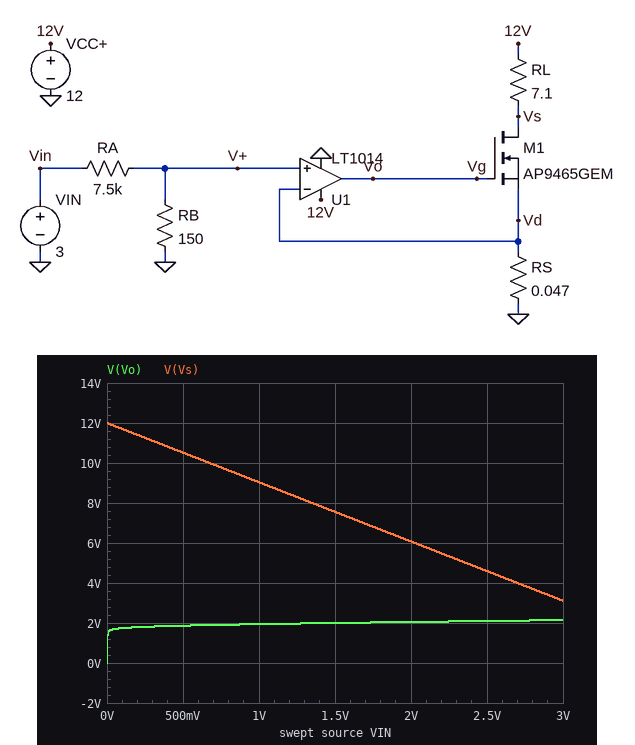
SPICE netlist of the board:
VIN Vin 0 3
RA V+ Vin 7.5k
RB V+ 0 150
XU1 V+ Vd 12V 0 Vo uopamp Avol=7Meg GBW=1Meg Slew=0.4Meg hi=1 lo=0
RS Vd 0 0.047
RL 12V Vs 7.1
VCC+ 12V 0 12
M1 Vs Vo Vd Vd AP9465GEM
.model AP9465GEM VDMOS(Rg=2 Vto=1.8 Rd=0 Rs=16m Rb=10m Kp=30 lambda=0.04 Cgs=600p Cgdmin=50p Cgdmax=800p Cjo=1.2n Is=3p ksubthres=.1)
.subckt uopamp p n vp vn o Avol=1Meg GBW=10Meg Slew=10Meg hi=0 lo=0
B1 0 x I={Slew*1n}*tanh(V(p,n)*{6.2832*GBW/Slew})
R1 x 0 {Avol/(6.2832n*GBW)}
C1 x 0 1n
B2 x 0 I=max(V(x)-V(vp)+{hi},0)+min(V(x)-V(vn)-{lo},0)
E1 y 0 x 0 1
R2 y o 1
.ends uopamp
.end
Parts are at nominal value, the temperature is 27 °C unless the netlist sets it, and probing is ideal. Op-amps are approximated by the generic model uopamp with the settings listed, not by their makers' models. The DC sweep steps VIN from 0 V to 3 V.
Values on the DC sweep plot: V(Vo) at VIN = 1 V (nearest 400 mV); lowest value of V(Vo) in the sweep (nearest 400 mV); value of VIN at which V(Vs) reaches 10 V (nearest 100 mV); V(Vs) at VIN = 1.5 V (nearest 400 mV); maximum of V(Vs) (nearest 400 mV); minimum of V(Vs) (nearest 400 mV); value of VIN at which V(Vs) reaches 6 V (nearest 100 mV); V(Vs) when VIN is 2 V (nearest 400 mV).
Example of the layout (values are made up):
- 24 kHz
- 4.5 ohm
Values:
- 2.0 V
- 0 V
- 700 mV
- 7.6 V
- 12.0 V
- 3.2 V
- 2.0 V
- 6.0 V
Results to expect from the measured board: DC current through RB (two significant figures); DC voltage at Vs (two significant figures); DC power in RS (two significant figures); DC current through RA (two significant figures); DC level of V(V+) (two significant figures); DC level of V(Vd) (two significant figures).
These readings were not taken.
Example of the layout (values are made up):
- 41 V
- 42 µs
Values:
- 390 µA
- 3.1 V
- 74 mW
- 390 µA
- 59 mV
- 59 mV
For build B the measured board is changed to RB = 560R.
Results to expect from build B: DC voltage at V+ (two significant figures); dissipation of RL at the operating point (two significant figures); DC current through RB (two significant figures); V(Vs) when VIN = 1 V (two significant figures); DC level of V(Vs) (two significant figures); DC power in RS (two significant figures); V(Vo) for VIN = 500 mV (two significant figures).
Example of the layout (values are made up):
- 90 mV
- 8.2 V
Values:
- 210 mV
- 20 W
- 370 µA
- 1.5 V
- 110 mV
- 130 mW
- 2.0 V
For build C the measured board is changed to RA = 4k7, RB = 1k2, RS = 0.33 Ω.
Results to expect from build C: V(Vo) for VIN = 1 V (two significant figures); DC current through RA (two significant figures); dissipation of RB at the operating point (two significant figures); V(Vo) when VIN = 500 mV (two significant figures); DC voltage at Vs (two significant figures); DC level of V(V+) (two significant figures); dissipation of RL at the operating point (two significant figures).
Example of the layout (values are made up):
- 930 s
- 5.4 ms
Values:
- 2.2 V
- 510 µA
- 310 µW
- 2.0 V
- 560 mV
- 610 mV
- 18 W
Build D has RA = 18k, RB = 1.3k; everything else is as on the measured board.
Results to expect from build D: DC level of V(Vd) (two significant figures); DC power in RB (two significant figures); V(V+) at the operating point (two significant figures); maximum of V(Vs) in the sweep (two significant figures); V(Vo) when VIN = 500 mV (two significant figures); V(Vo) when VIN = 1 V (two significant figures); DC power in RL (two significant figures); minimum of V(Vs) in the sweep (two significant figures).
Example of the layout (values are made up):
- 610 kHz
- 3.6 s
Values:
- 79 mV
- 31 µW
- 200 mV
- 12 V
- 2.0 V
- 2.2 V
- 20 W
- 110 mV
